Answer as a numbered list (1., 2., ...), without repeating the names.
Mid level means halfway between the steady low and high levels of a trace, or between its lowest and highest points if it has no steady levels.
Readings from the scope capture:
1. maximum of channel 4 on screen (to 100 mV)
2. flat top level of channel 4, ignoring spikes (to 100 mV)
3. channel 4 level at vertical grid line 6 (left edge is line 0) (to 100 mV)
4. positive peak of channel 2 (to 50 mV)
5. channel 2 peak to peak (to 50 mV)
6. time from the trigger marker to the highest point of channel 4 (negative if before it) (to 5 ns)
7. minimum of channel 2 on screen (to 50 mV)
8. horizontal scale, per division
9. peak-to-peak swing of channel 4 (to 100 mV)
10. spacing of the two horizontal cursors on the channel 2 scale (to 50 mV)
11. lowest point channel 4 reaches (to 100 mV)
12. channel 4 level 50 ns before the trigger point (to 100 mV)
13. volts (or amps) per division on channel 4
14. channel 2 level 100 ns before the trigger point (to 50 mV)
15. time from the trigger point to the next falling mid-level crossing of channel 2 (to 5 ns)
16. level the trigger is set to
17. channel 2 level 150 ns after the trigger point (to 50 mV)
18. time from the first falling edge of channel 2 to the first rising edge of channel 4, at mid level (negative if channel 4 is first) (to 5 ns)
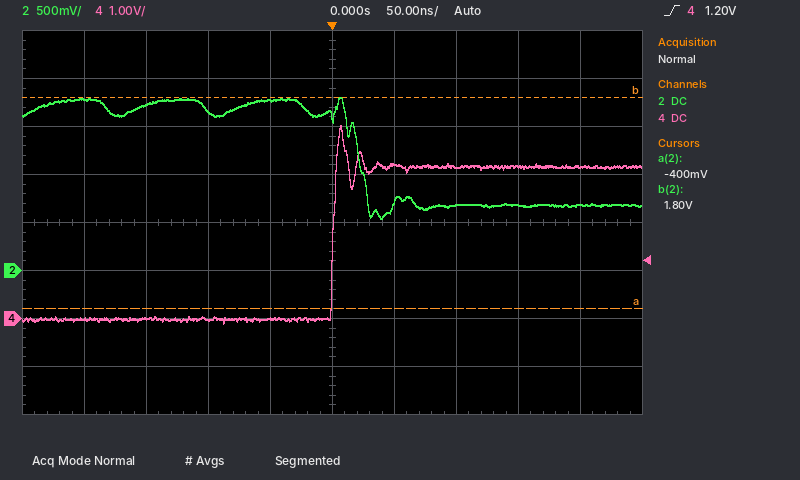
1. 4.0 V
2. 3.2 V
3. 3.2 V
4. 1.80 V
5. 1.25 V
6. +5 ns
7. 550 mV
8. 50 ns
9. 4.1 V
10. 2.20 V
11. -100 mV
12. 0.0 V
13. 1 V
14. 1.65 V
15. 20 ns
16. 1.20 V
17. 700 mV
18. -20 ns
